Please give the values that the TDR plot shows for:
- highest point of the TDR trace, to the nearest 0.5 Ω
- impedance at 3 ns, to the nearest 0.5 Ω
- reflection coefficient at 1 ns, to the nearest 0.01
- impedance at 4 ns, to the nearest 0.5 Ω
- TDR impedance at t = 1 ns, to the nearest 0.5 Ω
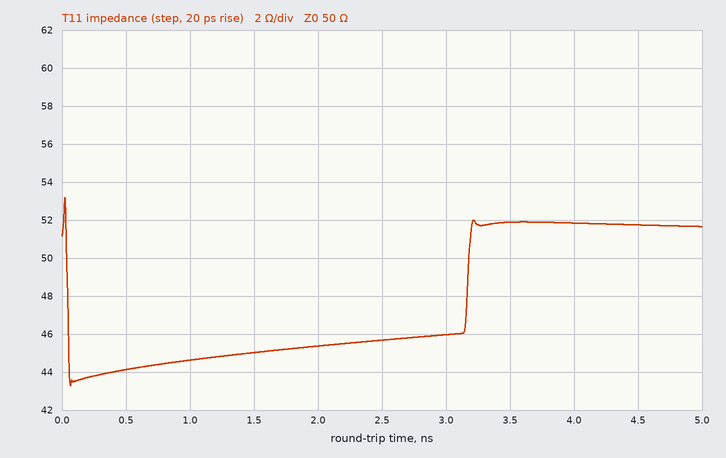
53.0 Ω
46.0 Ω
-0.06
52.0 Ω
44.5 Ω
